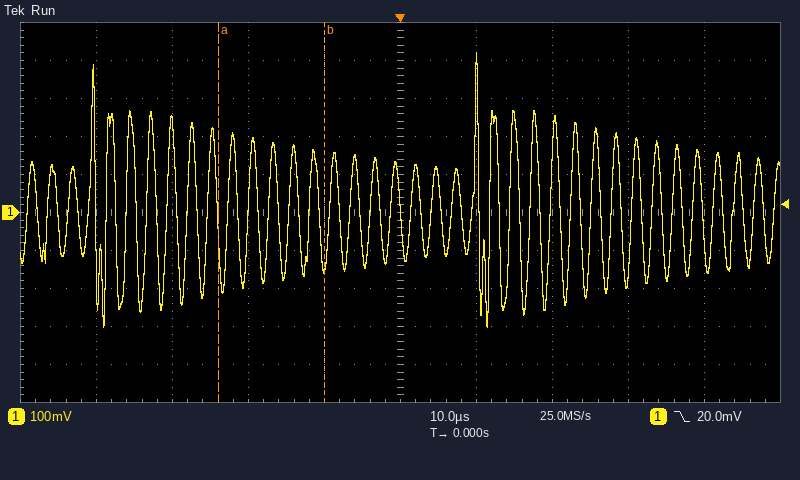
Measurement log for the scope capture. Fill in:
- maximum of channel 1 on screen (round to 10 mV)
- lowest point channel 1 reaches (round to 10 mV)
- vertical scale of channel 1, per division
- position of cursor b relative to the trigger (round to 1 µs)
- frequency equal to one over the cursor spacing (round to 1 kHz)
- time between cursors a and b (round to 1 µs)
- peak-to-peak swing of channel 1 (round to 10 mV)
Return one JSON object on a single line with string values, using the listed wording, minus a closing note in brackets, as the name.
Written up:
{"maximum of channel 1 on screen": "420 mV", "lowest point channel 1 reaches": "-300 mV", "vertical scale of channel 1, per division": "100 mV", "position of cursor b relative to the trigger": "-10 µs", "frequency equal to one over the cursor spacing": "71 kHz", "time between cursors a and b": "14 µs", "peak-to-peak swing of channel 1": "720 mV"}
